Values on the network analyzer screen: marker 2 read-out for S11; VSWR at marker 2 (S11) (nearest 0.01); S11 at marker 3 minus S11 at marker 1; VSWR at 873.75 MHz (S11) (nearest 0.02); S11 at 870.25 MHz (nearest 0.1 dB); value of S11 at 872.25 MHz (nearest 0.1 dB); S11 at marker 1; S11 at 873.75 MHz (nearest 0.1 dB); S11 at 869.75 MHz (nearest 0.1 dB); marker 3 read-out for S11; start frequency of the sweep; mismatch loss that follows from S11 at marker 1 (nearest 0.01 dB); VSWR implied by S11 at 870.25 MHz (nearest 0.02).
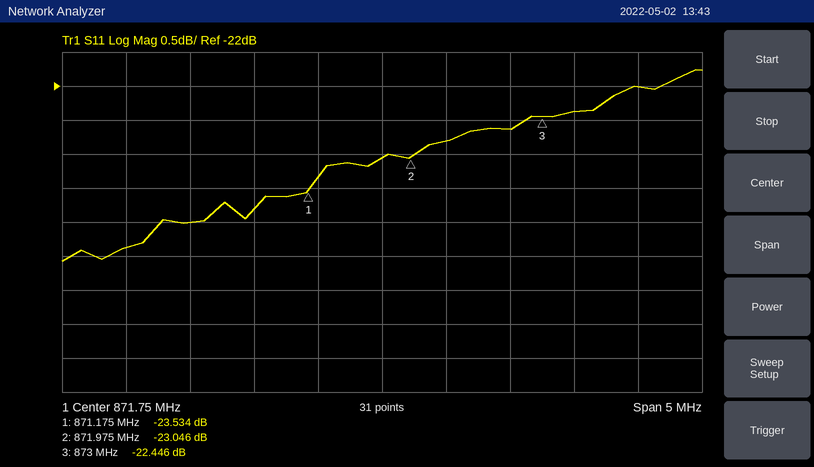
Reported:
-23.046 dB
1.15
1.088 dB
1.18
-24.0 dB
-22.8 dB
-23.534 dB
-22.0 dB
-24.4 dB
-22.446 dB
869.25 MHz
0.02 dB
1.14
